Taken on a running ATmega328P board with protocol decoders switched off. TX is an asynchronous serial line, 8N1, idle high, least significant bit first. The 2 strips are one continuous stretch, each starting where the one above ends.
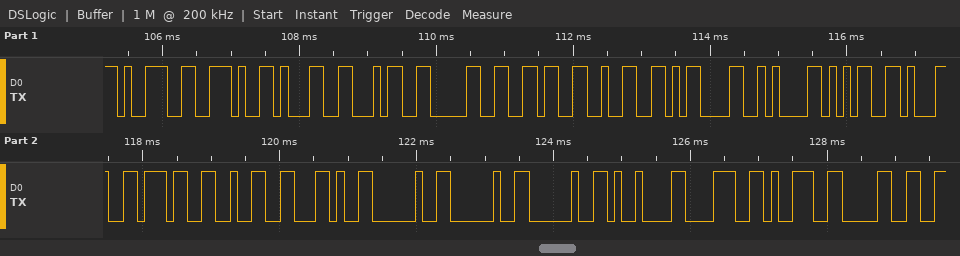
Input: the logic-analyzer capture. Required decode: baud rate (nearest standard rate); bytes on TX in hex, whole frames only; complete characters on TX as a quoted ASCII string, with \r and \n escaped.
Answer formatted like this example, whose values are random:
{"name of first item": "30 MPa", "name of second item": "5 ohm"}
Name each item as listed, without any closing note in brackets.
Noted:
{"baud rate": "9600 baud", "bytes on TX in hex, whole frames only": "39 2E 31 34 30 36 32 0D 0A 35 31 37 32 2C 20 20 20 09 38 39 30", "complete characters on TX as a quoted ASCII string, with \\r and \\n escaped": "\"9.14062\\r\\n5172,   \\t890\""}
